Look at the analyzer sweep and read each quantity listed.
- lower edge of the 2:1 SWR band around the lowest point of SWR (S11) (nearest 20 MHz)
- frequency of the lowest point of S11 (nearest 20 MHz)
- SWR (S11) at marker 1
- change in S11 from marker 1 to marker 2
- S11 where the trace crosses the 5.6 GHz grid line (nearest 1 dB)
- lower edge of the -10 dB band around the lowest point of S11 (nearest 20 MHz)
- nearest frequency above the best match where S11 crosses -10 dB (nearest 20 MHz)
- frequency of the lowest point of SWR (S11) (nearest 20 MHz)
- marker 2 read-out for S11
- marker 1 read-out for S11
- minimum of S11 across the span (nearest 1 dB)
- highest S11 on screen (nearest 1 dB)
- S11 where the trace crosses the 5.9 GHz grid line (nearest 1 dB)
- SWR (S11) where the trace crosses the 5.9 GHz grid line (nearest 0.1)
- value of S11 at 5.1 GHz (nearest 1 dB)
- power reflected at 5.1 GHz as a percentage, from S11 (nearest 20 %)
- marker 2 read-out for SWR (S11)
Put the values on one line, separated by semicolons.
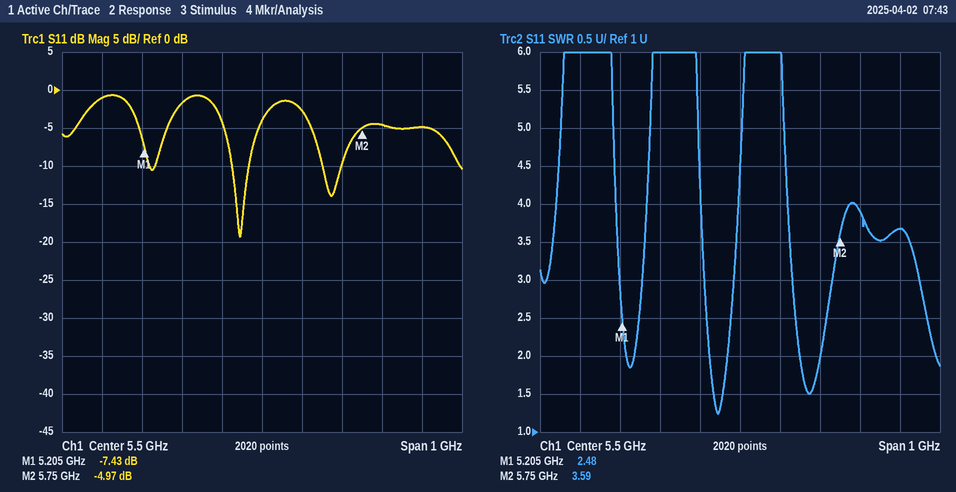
5.42 GHz; 5.44 GHz; 2.48; 2.46 dB; -3 dB; 5.42 GHz; 5.46 GHz; 5.44 GHz; -4.97 dB; -7.43 dB; -19 dB; -1 dB; -5 dB; 3.7; -1 dB; 80 %; 3.59
